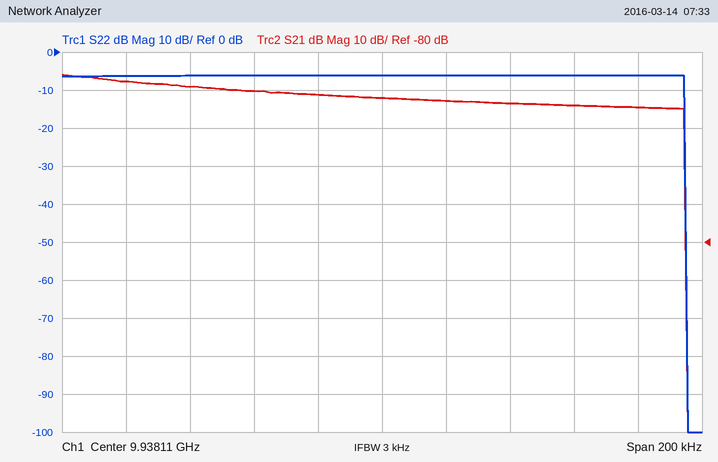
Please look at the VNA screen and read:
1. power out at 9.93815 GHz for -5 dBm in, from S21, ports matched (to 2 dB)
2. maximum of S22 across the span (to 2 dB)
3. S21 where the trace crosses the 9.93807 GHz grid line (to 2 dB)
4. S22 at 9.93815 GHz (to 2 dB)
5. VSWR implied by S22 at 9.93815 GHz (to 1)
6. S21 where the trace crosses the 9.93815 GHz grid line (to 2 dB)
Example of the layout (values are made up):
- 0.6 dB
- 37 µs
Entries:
- -48 dBm
- -6 dB
- -40 dB
- -6 dB
- 3
- -44 dB
